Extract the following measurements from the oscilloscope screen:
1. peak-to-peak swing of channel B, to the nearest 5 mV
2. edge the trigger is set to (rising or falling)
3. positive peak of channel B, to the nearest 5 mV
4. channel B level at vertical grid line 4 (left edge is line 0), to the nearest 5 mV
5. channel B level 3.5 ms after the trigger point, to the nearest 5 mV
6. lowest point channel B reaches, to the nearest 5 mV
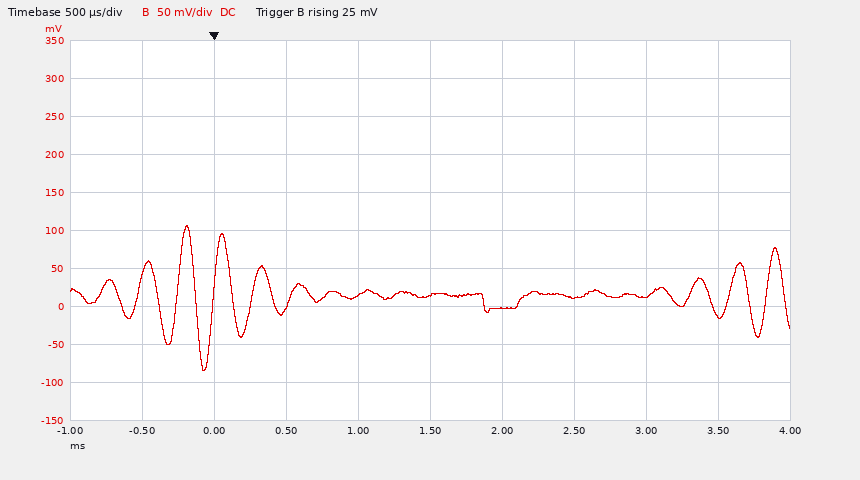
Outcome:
190 mV
rising
105 mV
15 mV
-10 mV
-85 mV
